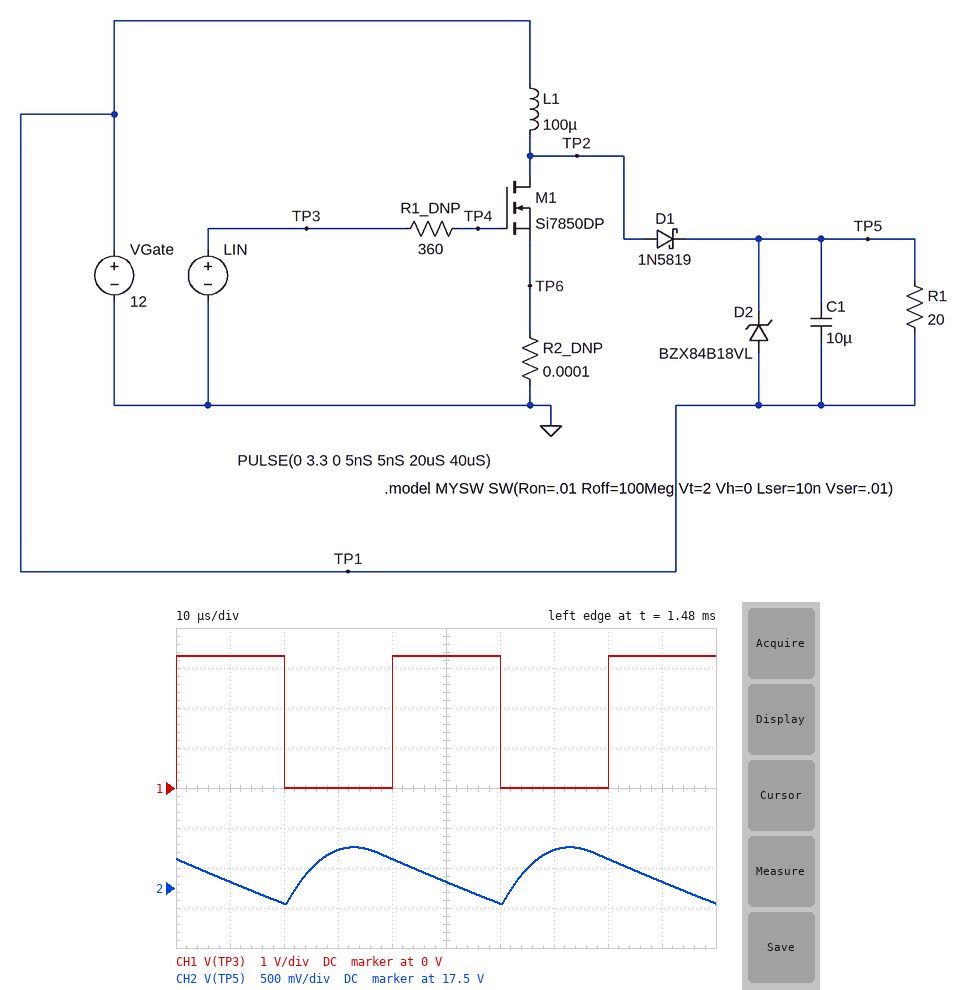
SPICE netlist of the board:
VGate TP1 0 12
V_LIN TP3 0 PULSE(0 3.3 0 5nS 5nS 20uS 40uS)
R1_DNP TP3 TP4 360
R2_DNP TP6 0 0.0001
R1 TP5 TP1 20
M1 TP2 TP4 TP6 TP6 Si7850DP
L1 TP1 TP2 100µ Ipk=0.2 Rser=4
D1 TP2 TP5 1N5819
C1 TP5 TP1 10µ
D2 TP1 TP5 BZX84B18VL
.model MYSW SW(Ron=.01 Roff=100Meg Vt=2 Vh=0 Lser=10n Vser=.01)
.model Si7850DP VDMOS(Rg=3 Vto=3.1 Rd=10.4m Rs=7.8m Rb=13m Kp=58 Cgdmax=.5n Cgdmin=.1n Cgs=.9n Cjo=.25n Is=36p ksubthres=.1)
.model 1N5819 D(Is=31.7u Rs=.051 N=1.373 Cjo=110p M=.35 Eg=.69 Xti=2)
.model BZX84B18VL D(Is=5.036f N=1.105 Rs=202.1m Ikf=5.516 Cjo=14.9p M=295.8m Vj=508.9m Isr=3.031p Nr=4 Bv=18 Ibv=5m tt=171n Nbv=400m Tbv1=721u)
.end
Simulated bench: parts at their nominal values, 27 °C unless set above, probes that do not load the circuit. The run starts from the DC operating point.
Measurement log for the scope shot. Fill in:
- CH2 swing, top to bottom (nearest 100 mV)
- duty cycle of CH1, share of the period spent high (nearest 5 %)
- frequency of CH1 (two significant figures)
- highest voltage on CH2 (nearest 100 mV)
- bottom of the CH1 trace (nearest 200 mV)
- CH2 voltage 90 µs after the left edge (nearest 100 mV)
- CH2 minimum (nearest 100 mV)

700 mV
50 %
25 kHz
18.0 V
0 V
17.6 V
17.3 V
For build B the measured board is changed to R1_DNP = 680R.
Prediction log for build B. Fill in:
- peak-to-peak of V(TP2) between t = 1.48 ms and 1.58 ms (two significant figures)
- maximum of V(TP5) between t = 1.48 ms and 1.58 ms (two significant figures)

16 V
17 V
